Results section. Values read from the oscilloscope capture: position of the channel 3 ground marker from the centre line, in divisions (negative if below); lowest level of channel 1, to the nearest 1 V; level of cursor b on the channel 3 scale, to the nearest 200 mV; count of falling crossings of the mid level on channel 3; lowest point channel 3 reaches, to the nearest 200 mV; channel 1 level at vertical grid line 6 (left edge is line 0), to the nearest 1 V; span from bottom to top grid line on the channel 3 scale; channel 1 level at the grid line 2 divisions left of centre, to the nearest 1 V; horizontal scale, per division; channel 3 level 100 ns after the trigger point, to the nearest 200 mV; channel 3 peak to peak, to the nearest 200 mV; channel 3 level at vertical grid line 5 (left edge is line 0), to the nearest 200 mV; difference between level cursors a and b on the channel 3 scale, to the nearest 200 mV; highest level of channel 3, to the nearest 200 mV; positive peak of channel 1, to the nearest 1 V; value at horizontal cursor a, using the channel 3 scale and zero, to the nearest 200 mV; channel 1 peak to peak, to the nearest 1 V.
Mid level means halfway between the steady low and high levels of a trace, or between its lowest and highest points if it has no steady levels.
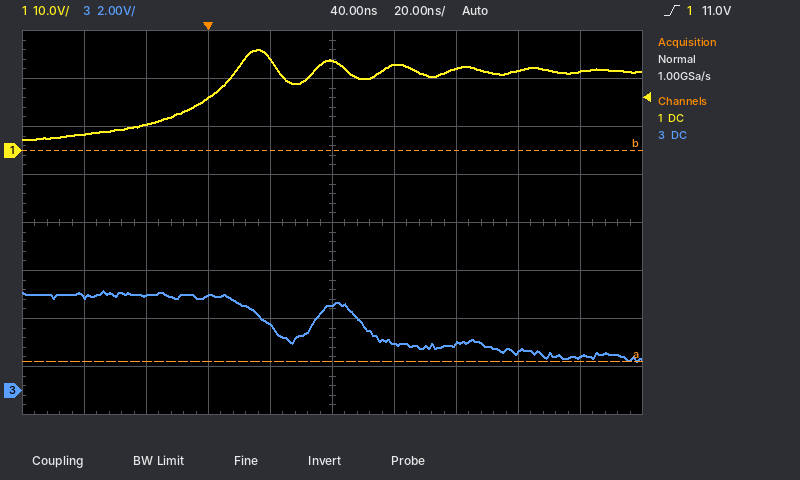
-3.5 div
2 V
10.0 V
2
1.2 V
18 V
16 V
11 V
20 ns
1.6 V
3.0 V
3.6 V
8.8 V
4.2 V
21 V
1.2 V
19 V
